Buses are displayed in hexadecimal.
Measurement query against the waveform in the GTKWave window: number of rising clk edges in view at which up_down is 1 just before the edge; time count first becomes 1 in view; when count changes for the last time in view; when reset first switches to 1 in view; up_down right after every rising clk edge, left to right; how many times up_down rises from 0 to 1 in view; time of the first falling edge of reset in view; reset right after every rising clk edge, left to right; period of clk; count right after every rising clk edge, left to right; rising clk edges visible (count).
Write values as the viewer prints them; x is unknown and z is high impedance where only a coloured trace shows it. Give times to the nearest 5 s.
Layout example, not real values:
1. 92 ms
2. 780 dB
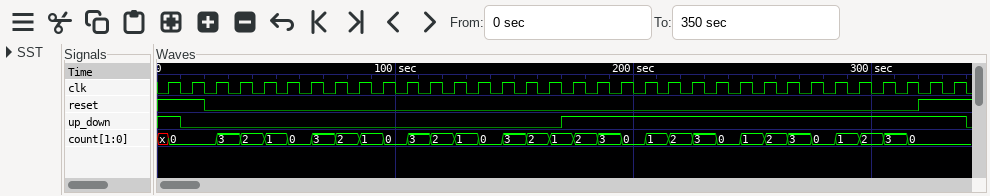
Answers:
1. 18
2. 45 s
3. 315 s
4. 320 s
5. 1 0 0 0 0 0 0 0 0 0 0 0 0 0 0 0 0 1 1 1 1 1 1 1 1 1 1 1 1 1 1 1 1 1
6. 1
7. 20 s
8. 1 1 0 0 0 0 0 0 0 0 0 0 0 0 0 0 0 0 0 0 0 0 0 0 0 0 0 0 0 0 0 0 1 1
9. 10 s
10. 0, 0, 3, 2, 1, 0, 3, 2, 1, 0, 3, 2, 1, 0, 3, 2, 1, 2, 3, 0, 1, 2, 3, 0, 1, 2, 3, 0, 1, 2, 3, 0, 0, 0
11. 34
